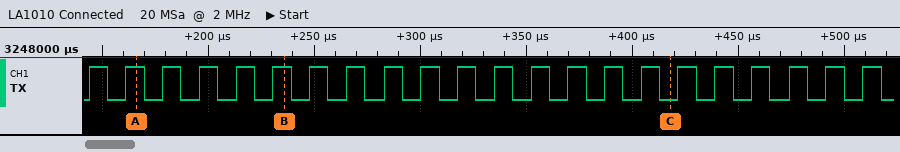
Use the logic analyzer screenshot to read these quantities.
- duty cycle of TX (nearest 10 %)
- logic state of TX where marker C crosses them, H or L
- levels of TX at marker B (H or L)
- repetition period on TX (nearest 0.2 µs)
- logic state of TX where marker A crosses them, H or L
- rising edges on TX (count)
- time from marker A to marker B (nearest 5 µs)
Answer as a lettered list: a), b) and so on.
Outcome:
a) 50 %
b) TX=L
c) TX=H
d) 17.4 µs
e) TX=H
f) 22
g) 70 µs
